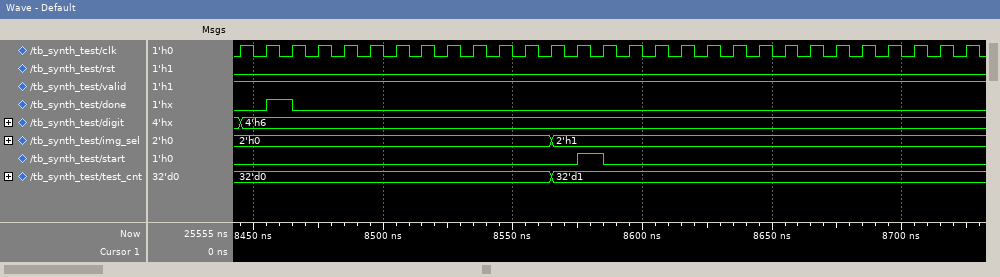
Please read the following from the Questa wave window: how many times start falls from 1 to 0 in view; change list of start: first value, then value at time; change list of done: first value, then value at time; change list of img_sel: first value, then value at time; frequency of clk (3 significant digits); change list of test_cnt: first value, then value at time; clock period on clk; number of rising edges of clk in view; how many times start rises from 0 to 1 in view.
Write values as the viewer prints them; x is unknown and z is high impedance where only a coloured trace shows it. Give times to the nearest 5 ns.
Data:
1
0, 1 at 8575 ns, 0 at 8585 ns
0, 1 at 8455 ns, 0 at 8465 ns
2'h0, 2'h1 at 8565 ns
100 MHz
32'd0, 32'd1 at 8565 ns
10 ns
29
1
